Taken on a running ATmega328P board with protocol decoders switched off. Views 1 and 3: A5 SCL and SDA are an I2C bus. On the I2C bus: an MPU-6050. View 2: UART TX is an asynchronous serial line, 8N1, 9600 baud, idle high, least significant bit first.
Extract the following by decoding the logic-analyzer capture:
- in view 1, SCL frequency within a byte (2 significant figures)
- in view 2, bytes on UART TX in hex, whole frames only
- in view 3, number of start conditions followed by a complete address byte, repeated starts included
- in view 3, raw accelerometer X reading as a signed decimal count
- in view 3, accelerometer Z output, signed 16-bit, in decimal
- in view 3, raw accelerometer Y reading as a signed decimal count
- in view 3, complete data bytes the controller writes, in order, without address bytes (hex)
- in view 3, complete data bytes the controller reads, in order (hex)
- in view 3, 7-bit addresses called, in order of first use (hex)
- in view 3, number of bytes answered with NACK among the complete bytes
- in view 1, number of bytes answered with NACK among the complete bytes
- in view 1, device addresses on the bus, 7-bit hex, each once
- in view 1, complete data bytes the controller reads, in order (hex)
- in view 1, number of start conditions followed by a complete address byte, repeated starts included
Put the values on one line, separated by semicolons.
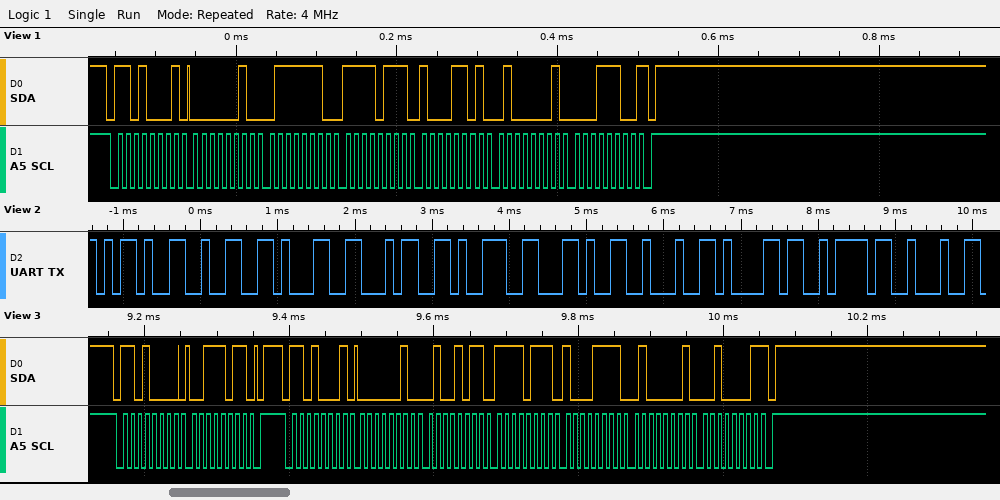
100 kHz; 2D 32 31 34 39 2C 22 61 7A 22; 2; 587; 16673; -2161; 3B; 02 4B F7 8F 41 21; 0x68; 1; 1; 0x68; 02 7E F7 8D 41 1C; 1
